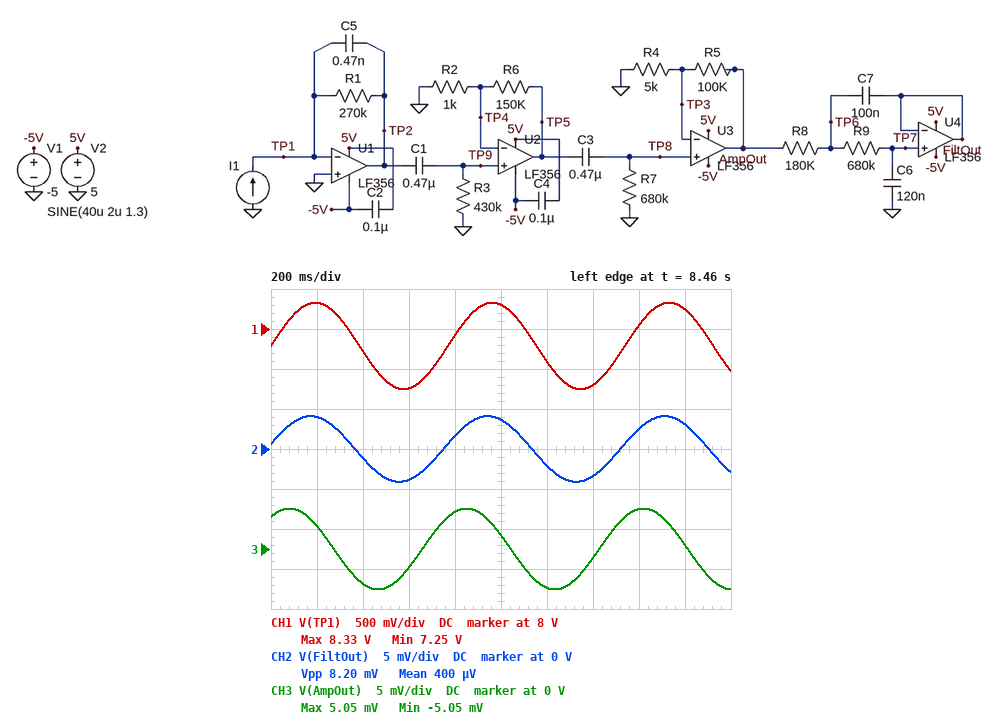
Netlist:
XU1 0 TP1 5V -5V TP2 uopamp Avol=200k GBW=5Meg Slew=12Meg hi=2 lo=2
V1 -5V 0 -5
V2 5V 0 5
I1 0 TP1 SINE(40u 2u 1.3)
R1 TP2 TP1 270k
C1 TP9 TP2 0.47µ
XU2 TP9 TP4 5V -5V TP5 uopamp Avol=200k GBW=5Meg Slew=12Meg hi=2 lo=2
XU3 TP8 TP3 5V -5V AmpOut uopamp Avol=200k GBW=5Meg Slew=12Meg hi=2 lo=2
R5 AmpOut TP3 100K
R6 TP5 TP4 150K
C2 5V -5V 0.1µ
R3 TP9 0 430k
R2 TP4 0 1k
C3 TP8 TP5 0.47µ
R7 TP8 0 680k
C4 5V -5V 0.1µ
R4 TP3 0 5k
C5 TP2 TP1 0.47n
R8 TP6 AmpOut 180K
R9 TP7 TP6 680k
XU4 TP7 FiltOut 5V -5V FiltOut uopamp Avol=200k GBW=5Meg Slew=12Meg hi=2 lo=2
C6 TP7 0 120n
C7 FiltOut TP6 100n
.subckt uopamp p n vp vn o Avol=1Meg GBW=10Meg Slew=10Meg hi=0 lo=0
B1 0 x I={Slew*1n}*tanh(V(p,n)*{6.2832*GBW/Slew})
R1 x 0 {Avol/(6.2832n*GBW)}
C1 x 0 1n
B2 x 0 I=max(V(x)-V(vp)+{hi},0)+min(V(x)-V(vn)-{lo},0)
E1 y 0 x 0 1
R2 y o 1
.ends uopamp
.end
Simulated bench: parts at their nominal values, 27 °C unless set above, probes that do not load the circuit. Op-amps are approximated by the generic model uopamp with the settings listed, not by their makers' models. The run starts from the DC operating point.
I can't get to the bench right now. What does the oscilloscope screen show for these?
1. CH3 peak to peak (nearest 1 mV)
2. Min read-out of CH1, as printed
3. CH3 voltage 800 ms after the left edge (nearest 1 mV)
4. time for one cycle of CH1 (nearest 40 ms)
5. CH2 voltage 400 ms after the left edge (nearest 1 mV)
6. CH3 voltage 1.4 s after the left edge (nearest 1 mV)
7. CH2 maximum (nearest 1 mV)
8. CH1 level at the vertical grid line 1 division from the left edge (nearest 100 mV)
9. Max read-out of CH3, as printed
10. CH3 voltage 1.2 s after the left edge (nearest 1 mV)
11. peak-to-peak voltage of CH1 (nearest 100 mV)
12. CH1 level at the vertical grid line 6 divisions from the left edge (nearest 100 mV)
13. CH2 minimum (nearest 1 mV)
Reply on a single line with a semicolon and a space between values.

10 mV; 7.25 V; 5 mV; 760 ms; -1 mV; -1 mV; 4 mV; 8.3 V; 5.05 mV; -5 mV; 1.1 V; 7.6 V; -4 mV
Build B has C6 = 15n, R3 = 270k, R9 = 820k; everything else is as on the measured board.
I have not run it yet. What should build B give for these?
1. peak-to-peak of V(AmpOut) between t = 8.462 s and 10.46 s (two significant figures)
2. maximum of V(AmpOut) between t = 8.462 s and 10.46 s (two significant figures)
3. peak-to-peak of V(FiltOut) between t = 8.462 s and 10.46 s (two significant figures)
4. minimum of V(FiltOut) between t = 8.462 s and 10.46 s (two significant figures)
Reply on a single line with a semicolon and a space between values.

8.5 mV; 4.3 mV; 8.6 mV; -4.3 mV
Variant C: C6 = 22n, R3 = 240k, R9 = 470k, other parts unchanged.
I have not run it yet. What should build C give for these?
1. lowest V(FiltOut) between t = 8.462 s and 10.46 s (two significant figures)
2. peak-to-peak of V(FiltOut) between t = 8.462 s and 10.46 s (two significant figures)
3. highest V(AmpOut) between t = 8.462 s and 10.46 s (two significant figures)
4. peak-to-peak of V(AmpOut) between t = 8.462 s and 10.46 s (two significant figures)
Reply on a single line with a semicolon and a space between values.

-4.0 mV; 8.1 mV; 4.0 mV; 8.0 mV
